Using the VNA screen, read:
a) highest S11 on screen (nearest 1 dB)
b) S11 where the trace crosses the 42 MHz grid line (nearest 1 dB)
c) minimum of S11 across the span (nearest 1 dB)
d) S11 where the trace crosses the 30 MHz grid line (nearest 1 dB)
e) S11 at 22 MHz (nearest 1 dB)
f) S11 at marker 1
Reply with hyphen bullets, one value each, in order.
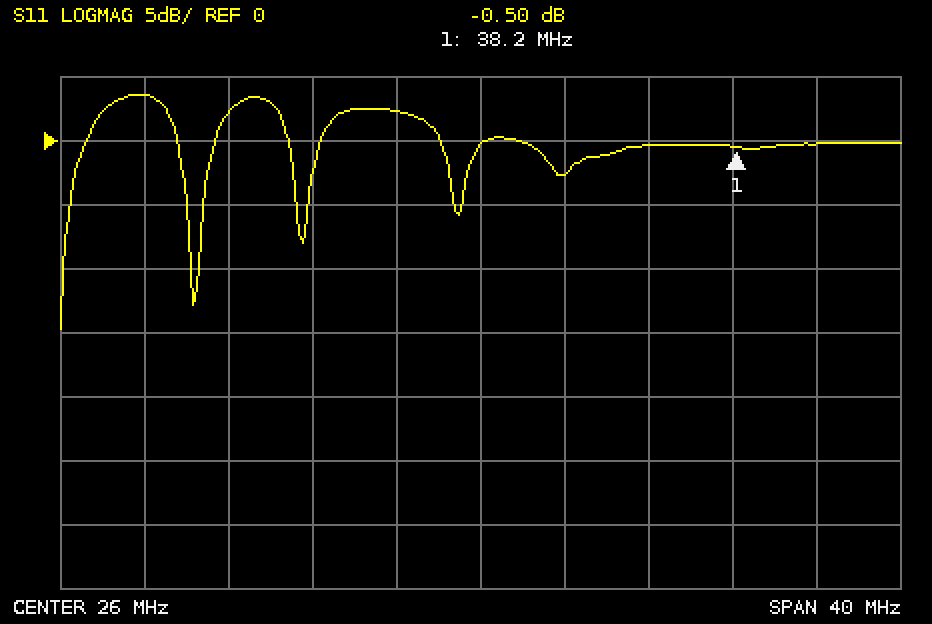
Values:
- 4 dB
- 0 dB
- -15 dB
- -3 dB
- 2 dB
- -0.50 dB
